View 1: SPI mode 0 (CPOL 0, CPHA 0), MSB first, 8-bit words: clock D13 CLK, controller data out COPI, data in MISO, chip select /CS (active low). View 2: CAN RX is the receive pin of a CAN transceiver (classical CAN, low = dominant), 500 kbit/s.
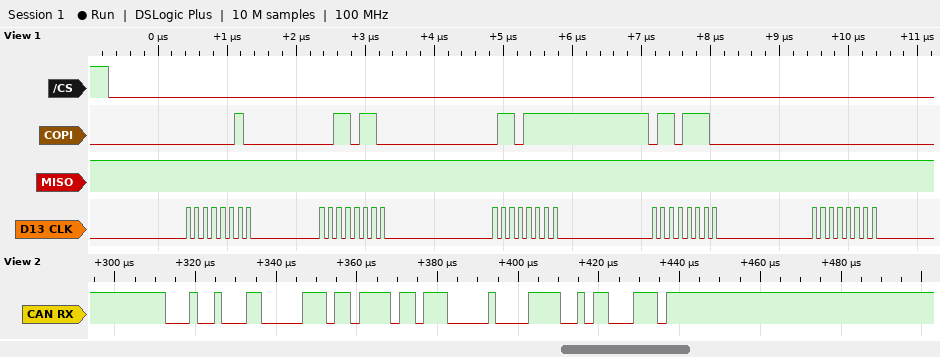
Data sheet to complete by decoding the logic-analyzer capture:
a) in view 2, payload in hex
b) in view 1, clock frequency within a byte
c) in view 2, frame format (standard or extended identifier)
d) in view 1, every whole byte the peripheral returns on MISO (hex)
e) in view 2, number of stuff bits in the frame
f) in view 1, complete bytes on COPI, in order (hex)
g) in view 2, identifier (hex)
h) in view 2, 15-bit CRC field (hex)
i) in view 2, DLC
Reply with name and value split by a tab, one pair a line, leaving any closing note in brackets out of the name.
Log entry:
in view 2, payload in hex	6F 6E 00
in view 1, clock frequency within a byte	8 MHz
in view 2, frame format	standard
in view 1, every whole byte the peripheral returns on MISO	FF FF FF FF FF
in view 2, number of stuff bits in the frame	2
in view 1, complete bytes on COPI, in order	02 36 6F 6E 00
in view 2, identifier	0x123
in view 2, 15-bit CRC field	0x7963
in view 2, DLC	3
